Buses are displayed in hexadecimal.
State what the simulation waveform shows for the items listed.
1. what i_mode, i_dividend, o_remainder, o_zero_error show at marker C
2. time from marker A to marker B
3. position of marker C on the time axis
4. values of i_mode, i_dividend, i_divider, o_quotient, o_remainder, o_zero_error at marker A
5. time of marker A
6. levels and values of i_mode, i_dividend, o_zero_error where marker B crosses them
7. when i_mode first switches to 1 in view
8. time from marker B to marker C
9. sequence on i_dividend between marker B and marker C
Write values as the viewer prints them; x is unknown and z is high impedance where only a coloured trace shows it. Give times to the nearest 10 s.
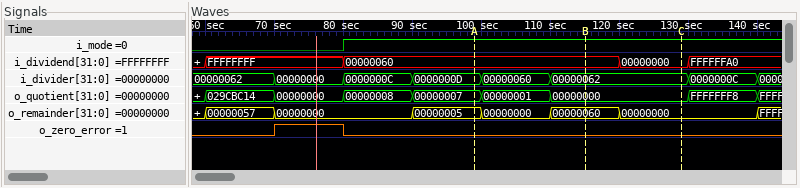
i_mode=1, i_dividend=00000000, o_remainder=00000000, o_zero_error=0
20 s
130 s
i_mode=1, i_dividend=00000060, i_divider=0000000D, o_quotient=00000007, o_remainder=00000005, o_zero_error=0
100 s
i_mode=1, i_dividend=00000060, o_zero_error=0
80 s
10 s
00000060, 00000000
